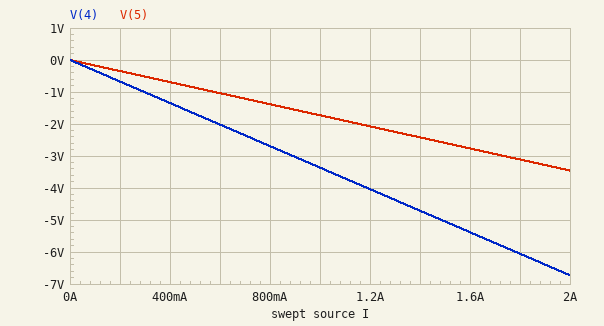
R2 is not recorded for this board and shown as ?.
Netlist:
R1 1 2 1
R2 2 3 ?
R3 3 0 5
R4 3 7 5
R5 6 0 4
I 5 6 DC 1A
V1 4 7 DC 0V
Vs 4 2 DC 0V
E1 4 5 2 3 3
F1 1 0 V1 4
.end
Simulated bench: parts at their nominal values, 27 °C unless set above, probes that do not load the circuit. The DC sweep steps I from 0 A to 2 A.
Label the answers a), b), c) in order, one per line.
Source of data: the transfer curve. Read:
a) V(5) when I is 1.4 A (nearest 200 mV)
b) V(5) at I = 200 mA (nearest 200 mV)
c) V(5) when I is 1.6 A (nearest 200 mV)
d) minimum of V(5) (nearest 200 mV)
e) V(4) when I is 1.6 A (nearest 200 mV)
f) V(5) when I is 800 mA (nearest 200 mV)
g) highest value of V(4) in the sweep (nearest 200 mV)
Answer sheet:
a) -2.4 V
b) -400 mV
c) -2.8 V
d) -3.4 V
e) -5.4 V
f) -1.4 V
g) 0 V
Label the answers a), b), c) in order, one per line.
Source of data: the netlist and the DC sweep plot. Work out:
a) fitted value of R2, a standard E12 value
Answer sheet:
a) 1.2 Ω
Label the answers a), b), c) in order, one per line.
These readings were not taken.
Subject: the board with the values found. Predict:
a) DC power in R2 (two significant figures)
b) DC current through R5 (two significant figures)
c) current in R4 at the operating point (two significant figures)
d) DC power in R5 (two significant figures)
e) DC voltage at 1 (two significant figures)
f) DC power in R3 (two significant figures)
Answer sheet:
a) 250 mW
b) 1.0 A
c) 110 mA
d) 4.0 W
e) -2.9 V
f) 1.6 W
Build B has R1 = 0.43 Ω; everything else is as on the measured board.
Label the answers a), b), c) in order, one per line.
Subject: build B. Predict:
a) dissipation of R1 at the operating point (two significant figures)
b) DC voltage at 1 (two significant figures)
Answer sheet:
a) 82 mW
b) -3.2 V
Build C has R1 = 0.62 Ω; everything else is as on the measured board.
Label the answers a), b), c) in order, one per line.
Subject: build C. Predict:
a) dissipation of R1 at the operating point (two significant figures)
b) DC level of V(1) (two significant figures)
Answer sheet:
a) 120 mW
b) -3.1 V
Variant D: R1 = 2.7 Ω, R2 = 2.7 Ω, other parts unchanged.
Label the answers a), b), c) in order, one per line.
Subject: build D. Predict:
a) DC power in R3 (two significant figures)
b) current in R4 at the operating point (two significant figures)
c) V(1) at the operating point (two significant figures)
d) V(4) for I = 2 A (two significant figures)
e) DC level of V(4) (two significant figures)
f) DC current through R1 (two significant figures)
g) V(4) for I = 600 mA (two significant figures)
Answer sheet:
a) 870 mW
b) 150 mA
c) -1.2 V
d) -5.6 V
e) -2.8 V
f) 580 mA
g) -1.7 V
